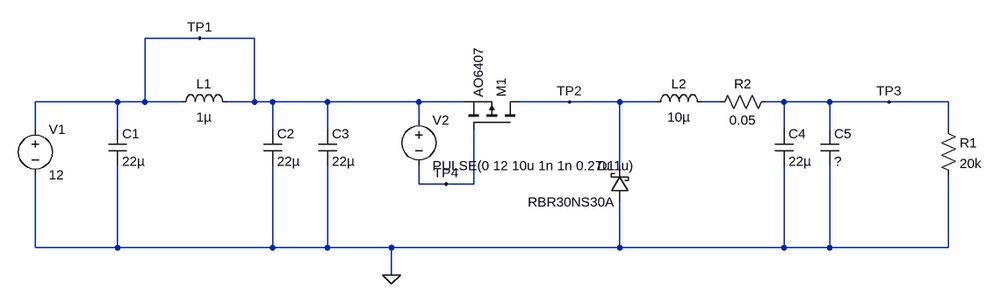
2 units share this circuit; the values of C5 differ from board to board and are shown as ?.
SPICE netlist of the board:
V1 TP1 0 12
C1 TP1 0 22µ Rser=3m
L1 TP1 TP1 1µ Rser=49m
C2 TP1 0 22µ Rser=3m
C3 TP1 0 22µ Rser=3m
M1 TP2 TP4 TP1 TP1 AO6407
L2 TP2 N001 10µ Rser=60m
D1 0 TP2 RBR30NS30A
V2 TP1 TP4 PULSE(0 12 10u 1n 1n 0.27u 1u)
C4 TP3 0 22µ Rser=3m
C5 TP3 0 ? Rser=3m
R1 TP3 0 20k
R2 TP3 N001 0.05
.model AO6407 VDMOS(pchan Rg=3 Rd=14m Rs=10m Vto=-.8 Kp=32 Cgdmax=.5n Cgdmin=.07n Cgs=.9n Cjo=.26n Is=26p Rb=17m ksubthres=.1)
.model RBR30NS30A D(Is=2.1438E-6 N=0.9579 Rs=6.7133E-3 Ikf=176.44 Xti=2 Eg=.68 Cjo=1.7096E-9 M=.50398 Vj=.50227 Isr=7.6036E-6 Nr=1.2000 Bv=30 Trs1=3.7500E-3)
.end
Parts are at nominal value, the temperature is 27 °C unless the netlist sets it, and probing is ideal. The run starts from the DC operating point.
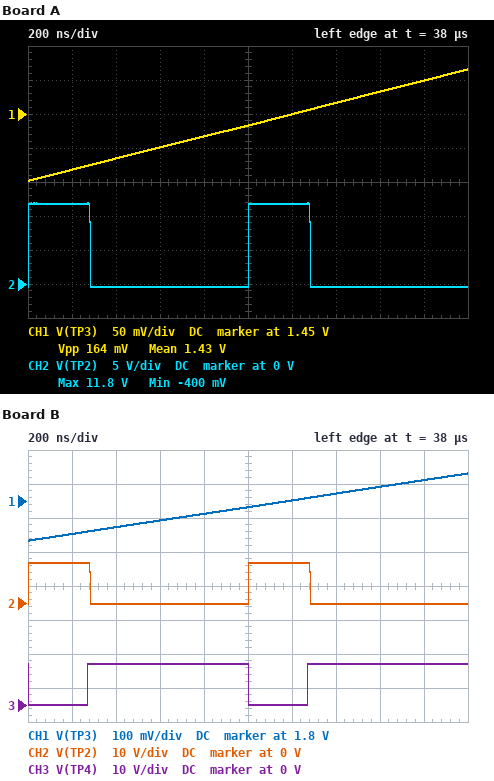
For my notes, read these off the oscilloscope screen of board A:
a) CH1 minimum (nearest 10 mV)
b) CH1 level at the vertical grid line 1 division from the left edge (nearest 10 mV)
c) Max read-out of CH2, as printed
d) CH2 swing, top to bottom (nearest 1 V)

1.35 V
1.37 V
11.8 V
12 V
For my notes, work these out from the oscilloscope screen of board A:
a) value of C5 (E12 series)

56 µF
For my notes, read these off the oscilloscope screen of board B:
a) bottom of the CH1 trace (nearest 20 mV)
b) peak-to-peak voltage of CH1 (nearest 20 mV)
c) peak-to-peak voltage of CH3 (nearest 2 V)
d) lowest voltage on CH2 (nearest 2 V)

1.68 V
200 mV
12 V
0 V
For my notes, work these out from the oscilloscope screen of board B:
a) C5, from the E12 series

39 µF
